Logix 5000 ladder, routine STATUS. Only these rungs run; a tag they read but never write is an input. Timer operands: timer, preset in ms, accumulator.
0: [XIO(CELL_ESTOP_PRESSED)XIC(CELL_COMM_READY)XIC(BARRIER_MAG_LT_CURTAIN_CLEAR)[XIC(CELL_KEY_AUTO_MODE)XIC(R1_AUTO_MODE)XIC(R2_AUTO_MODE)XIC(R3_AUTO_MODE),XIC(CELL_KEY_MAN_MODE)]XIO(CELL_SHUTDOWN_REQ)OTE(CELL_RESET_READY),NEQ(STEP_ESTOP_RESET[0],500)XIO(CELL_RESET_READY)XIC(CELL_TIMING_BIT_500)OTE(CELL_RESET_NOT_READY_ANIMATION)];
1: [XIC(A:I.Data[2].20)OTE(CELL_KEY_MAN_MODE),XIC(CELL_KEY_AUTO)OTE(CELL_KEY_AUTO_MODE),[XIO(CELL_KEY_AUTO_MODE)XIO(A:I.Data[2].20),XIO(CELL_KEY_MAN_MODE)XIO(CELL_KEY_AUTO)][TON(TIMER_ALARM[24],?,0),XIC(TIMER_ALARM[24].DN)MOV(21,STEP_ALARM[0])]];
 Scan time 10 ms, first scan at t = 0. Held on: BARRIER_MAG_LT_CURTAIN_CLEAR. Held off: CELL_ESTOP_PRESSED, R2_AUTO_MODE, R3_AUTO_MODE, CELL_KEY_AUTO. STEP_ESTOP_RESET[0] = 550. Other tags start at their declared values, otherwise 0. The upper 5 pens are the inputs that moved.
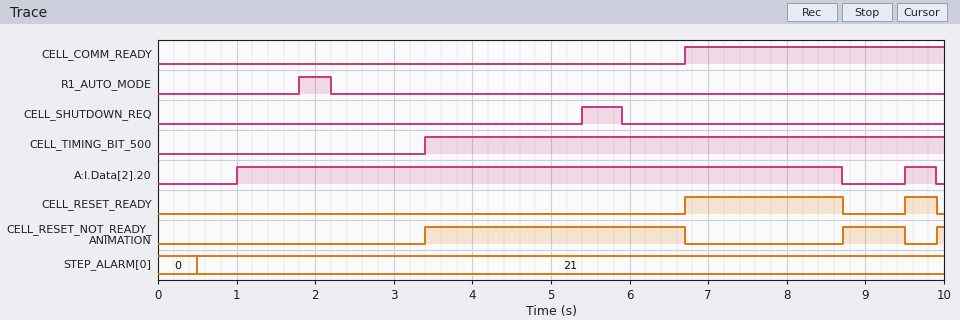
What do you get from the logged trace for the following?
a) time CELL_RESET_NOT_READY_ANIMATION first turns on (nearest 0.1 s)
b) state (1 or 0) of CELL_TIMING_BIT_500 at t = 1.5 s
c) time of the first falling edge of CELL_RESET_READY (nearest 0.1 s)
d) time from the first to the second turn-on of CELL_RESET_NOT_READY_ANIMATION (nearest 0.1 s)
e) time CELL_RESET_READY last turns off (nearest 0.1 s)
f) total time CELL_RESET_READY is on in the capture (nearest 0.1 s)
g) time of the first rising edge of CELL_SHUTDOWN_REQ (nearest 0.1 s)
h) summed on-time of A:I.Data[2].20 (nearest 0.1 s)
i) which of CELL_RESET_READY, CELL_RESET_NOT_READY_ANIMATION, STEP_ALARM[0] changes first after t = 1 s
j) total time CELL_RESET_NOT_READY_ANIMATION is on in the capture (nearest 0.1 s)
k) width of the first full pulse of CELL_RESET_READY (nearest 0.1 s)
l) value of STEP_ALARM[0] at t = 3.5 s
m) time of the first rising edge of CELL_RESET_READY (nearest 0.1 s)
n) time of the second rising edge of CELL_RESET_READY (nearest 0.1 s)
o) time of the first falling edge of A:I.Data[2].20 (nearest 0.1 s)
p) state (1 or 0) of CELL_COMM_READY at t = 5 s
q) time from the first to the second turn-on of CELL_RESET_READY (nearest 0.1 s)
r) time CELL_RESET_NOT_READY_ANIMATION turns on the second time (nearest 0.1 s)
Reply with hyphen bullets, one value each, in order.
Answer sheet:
- 3.4 s
- 0
- 8.7 s
- 5.3 s
- 9.9 s
- 2.4 s
- 5.4 s
- 8.1 s
- CELL_RESET_NOT_READY_ANIMATION
- 4.2 s
- 2.0 s
- 21
- 6.7 s
- 9.5 s
- 8.7 s
- 0
- 2.8 s
- 8.7 s
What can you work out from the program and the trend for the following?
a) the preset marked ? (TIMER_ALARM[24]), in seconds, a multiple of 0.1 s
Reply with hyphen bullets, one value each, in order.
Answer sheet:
- 0.5 s
